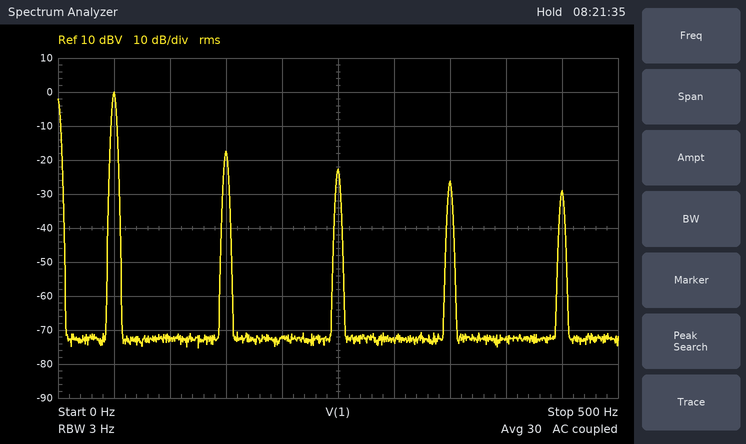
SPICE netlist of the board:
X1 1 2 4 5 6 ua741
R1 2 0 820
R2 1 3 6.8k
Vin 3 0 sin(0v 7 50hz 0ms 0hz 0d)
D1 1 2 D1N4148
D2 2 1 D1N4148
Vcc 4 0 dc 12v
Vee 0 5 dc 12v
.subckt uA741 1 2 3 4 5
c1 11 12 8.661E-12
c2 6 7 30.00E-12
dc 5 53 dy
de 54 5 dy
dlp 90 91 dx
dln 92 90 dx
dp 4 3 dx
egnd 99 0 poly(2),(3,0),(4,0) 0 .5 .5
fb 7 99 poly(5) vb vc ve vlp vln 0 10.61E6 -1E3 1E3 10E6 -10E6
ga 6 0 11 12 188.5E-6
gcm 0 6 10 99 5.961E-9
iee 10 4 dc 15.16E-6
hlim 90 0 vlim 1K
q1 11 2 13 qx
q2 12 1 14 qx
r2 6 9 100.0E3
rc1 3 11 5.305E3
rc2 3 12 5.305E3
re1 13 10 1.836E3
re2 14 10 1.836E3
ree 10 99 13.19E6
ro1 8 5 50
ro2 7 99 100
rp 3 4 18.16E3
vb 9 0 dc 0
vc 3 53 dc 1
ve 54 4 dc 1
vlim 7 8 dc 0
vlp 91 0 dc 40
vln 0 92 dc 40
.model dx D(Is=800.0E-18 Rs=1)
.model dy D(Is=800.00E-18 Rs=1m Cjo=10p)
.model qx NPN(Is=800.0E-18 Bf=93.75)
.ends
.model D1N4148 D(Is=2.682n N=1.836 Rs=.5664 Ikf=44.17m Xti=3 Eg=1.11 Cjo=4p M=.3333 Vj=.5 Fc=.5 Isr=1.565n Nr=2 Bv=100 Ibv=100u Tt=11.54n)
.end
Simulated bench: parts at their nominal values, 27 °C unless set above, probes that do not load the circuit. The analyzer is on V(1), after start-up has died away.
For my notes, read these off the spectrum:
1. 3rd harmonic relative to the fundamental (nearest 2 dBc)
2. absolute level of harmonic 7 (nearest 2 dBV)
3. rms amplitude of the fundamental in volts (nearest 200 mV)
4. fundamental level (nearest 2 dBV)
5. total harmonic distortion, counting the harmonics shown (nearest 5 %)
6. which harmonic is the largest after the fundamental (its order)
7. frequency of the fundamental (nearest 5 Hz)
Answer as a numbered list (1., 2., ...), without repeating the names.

1. -18 dBc
2. -26 dBV
3. 1.0 V
4. 0 dBV
5. 15 %
6. 3
7. 50 Hz
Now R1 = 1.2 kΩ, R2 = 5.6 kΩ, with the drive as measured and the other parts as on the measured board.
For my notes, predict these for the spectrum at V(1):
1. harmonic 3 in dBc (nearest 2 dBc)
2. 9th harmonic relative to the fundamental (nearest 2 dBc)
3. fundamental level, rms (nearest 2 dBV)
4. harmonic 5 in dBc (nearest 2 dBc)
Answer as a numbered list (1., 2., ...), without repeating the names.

1. -20 dBc
2. -32 dBc
3. 2 dBV
4. -26 dBc
